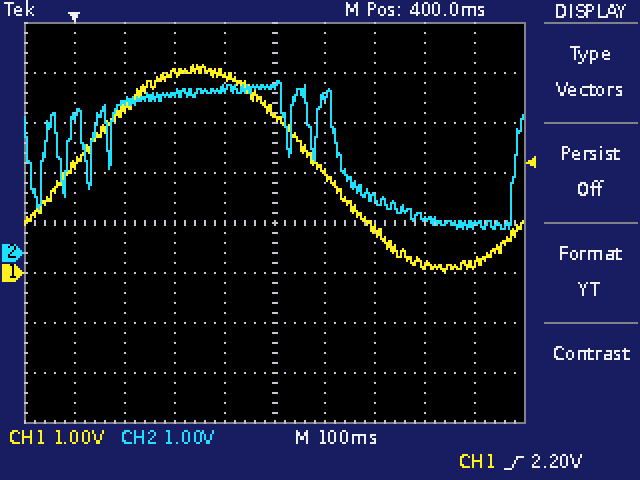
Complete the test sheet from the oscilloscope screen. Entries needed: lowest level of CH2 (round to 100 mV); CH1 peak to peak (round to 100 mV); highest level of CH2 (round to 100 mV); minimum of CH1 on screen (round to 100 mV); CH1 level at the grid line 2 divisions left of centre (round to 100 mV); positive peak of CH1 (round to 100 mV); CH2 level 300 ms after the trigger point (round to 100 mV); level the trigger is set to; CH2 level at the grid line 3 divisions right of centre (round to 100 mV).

500 mV
4.2 V
3.4 V
0.0 V
4.0 V
4.2 V
3.3 V
2.20 V
700 mV
